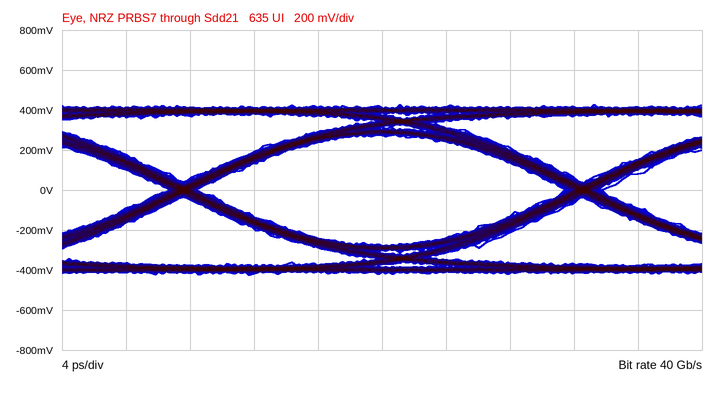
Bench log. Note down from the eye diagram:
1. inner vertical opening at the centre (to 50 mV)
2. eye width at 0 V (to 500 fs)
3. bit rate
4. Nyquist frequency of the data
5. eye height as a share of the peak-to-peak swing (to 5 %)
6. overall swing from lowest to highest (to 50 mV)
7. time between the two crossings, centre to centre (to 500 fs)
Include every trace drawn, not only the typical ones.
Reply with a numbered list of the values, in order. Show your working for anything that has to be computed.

1. 550 mV
2. 23.0 ps
3. 40 Gb/s
4. 20 GHz
5. 550 mV / 850 mV ≈ 65 %
6. 850 mV
7. 25.0 ps
